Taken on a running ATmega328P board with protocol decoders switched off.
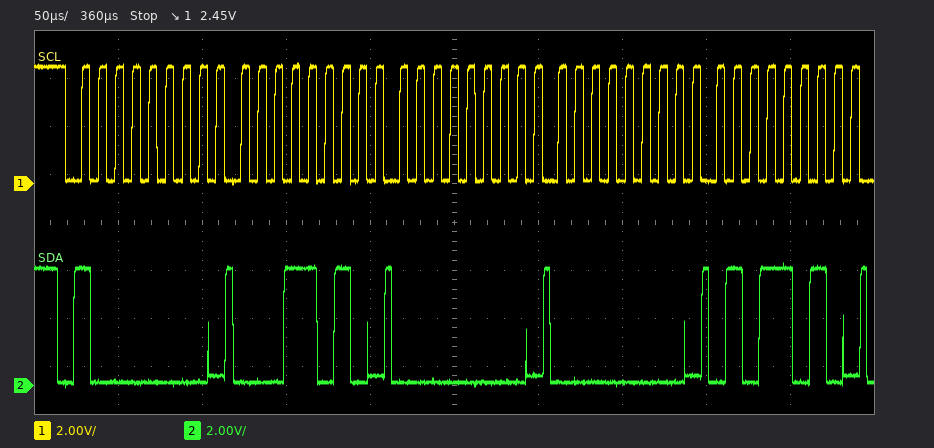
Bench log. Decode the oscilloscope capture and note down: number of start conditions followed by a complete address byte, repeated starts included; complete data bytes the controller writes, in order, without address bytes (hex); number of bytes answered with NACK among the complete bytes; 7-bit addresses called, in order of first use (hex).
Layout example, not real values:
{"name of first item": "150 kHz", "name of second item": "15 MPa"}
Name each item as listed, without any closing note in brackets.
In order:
{"number of start conditions followed by a complete address byte, repeated starts included": "1", "complete data bytes the controller writes, in order, without address bytes": "1A 00 00 5A", "number of bytes answered with NACK among the complete bytes": "0", "7-bit addresses called, in order of first use": "0x40"}
